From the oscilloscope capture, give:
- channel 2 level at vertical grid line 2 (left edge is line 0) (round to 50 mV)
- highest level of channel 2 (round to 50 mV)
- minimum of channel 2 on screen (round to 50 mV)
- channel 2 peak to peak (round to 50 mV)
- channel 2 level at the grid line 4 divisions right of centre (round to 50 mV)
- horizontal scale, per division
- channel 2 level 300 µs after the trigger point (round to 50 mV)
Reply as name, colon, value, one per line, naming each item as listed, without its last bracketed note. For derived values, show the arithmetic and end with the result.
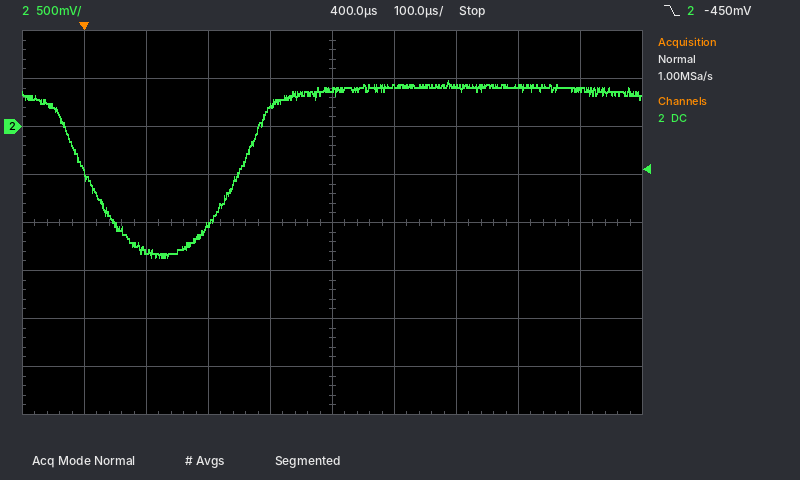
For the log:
channel 2 level at vertical grid line 2 (left edge is line 0): -1.30 V
highest level of channel 2: 500 mV
minimum of channel 2 on screen: -1.35 V
channel 2 peak to peak: 500 mV − (-1.35 V) = 1.85 V
channel 2 level at the grid line 4 divisions right of centre: 400 mV
horizontal scale, per division: 100 µs
channel 2 level 300 µs after the trigger point: 200 mV
